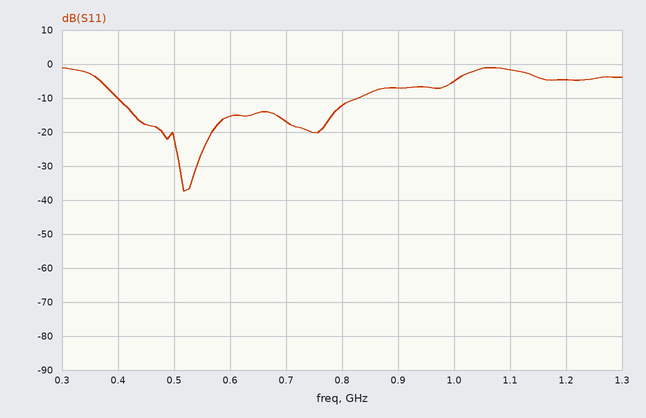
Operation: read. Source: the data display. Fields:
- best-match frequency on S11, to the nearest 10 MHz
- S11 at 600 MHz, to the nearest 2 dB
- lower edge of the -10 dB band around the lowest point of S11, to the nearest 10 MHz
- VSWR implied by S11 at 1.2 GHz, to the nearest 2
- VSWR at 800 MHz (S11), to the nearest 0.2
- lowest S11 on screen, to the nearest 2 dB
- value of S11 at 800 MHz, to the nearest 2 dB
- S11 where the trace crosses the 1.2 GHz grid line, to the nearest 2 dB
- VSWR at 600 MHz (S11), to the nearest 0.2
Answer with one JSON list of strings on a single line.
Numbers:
["520 MHz", "-16 dB", "400 MHz", "4", "1.6", "-38 dB", "-12 dB", "-4 dB", "1.4"]
